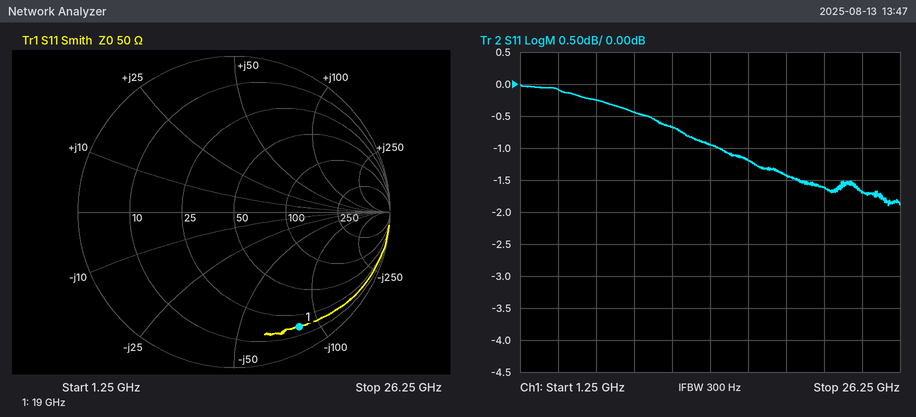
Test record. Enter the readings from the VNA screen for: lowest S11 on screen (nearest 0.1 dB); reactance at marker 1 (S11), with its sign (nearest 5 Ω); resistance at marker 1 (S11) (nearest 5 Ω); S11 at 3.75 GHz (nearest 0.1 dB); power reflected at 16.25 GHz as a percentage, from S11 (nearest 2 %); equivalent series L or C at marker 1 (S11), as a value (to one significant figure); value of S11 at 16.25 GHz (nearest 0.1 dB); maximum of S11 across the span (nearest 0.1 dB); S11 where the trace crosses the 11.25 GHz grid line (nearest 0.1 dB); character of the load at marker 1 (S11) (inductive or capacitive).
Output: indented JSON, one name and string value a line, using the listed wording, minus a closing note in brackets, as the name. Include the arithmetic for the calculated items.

{
  "lowest S11 on screen": "-1.9 dB",
  "reactance at marker 1 (S11), with its sign": "-85 Ω",
  "resistance at marker 1 (S11)": "15 Ω",
  "S11 at 3.75 GHz": "-0.1 dB",
  "power reflected at 16.25 GHz as a percentage, from S11": "10^(-1.2/10) ≈ 76 %",
  "equivalent series L or C at marker 1 (S11), as a value": "C = 1/(2π × 19 GHz × 85 Ω) ≈ 98.5 fF, so 100 fF to one significant figure",
  "value of S11 at 16.25 GHz": "-1.2 dB",
  "maximum of S11 across the span": "0.0 dB",
  "S11 where the trace crosses the 11.25 GHz grid line": "-0.7 dB",
  "character of the load at marker 1 (S11)": "capacitive"
}
